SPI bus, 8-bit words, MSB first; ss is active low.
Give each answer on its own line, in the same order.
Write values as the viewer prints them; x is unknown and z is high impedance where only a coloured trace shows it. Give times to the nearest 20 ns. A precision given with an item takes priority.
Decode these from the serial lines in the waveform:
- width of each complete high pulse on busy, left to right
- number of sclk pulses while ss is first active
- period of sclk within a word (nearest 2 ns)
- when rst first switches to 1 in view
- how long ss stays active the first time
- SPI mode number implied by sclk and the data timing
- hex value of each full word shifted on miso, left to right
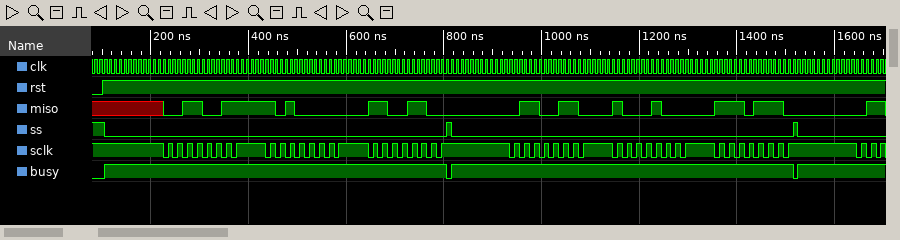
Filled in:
700 ns, 700 ns
24
20 ns
100 ns
700 ns
3
33, A0, CC, 66, 88, EE
